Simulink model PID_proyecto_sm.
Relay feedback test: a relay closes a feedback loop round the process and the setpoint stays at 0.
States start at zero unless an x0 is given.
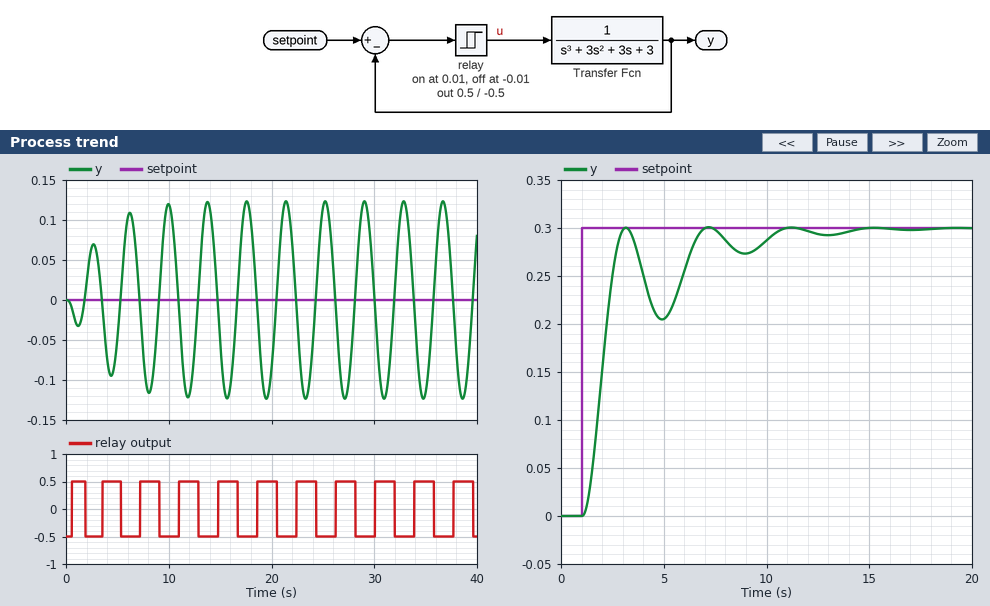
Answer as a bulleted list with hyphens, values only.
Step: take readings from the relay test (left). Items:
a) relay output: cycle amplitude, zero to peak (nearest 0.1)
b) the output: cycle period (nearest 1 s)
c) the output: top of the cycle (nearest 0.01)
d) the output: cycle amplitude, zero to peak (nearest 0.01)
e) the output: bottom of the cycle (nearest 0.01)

- 0.5
- 4 s
- 0.12
- 0.12
- -0.12
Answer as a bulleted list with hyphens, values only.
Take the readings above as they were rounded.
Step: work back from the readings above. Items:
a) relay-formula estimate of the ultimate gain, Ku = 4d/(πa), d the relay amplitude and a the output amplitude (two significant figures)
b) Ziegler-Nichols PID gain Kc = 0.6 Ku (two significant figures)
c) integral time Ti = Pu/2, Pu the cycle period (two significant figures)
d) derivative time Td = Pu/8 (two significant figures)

- 5.3
- 3.2
- 2.0 s
- 0.50 s
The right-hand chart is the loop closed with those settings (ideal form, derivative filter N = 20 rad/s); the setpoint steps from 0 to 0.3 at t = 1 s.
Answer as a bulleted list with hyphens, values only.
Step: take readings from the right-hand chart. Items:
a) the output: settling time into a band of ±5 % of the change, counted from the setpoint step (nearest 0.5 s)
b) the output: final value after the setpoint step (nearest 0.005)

- 9.0 s
- 0.300
